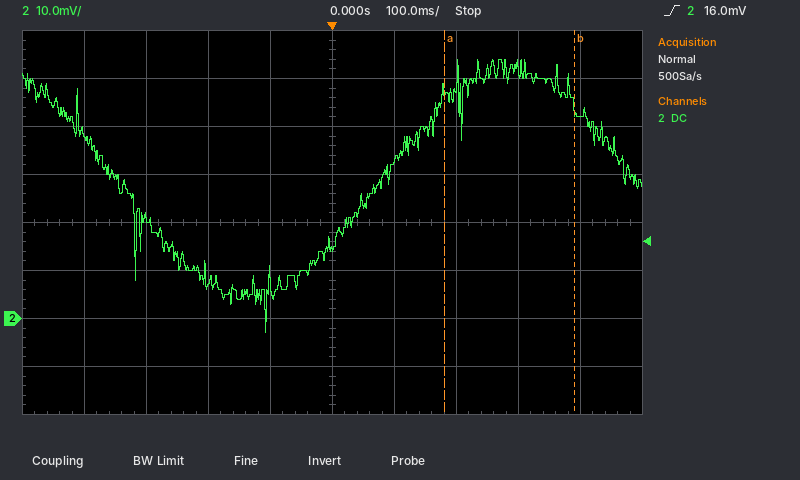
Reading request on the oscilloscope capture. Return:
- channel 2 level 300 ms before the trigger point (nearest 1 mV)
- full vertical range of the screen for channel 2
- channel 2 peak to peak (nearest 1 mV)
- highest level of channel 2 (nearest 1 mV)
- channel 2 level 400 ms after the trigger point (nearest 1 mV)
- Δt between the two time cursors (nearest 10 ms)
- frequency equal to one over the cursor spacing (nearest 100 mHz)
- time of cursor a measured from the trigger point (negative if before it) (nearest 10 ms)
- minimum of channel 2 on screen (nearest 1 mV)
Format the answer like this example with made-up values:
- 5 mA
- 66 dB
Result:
- 21 mV
- 80 mV
- 57 mV
- 54 mV
- 42 mV
- 210 ms
- 4.8 Hz
- +180 ms
- -3 mV
